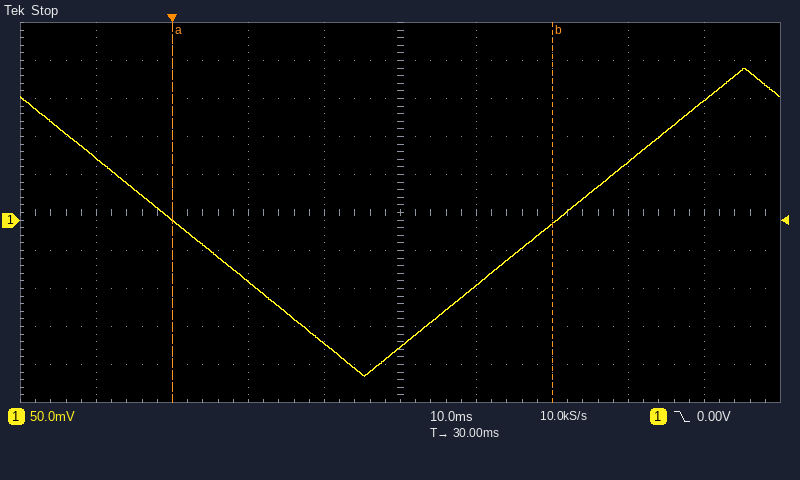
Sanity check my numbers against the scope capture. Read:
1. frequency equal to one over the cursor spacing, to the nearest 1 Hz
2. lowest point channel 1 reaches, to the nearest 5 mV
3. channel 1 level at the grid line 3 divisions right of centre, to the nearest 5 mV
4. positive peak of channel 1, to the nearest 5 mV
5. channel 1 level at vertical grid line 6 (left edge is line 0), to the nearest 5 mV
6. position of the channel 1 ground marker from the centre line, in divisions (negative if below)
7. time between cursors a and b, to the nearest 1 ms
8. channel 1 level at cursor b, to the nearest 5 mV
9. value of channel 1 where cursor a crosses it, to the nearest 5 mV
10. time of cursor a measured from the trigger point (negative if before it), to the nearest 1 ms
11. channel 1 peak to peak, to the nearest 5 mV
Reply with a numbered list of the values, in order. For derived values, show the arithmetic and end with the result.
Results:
1. 1 / 50 ms ≈ 20 Hz
2. -205 mV
3. 75 mV
4. 200 mV
5. -85 mV
6. -0.2 div
7. 50 ms
8. -5 mV
9. 0 mV
10. 0 ms
11. 200 mV − (-205 mV) = 405 mV
